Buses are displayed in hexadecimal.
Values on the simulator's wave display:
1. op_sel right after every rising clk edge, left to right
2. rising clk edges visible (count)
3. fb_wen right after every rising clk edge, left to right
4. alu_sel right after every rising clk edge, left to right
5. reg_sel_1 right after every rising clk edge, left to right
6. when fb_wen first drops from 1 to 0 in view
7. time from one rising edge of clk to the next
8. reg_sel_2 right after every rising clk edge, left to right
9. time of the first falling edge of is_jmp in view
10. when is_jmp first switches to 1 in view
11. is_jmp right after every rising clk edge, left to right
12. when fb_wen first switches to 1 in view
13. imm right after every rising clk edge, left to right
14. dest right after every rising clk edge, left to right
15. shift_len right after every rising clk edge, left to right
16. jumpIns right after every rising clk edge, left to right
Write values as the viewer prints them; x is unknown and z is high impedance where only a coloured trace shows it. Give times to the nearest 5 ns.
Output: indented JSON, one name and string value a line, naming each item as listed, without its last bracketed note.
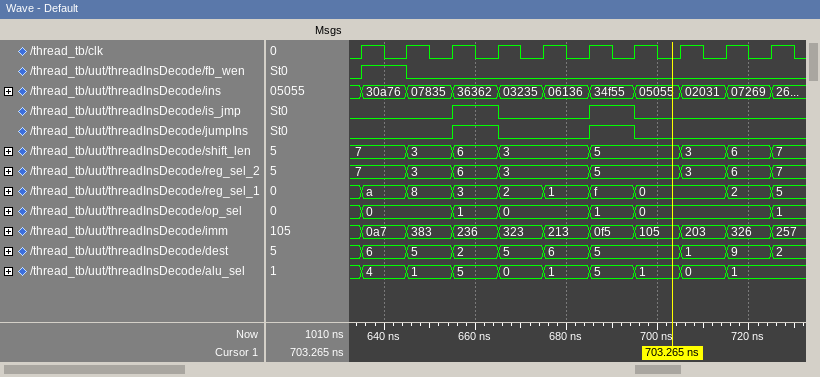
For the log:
{
  "op_sel right after every rising clk edge, left to right": "0, 0, 1, 0, 0, 1, 0, 0, 0, 1",
  "rising clk edges visible": "10",
  "fb_wen right after every rising clk edge, left to right": "1 0 0 0 0 0 0 0 0 0",
  "alu_sel right after every rising clk edge, left to right": "4, 1, 5, 0, 1, 5, 1, 0, 1, 1",
  "reg_sel_1 right after every rising clk edge, left to right": "a, 8, 3, 2, 1, f, 0, 0, 2, 5",
  "when fb_wen first drops from 1 to 0 in view": "645 ns",
  "time from one rising edge of clk to the next": "10 ns",
  "reg_sel_2 right after every rising clk edge, left to right": "7, 3, 6, 3, 3, 5, 5, 3, 6, 7",
  "time of the first falling edge of is_jmp in view": "665 ns",
  "when is_jmp first switches to 1 in view": "655 ns",
  "is_jmp right after every rising clk edge, left to right": "0 0 1 0 0 1 0 0 0 0",
  "when fb_wen first switches to 1 in view": "635 ns",
  "imm right after every rising clk edge, left to right": "0a7, 383, 236, 323, 213, 0f5, 105, 203, 326, 257",
  "dest right after every rising clk edge, left to right": "6, 5, 2, 5, 6, 5, 5, 1, 9, 2",
  "shift_len right after every rising clk edge, left to right": "7, 3, 6, 3, 3, 5, 5, 3, 6, 7",
  "jumpIns right after every rising clk edge, left to right": "0 0 1 0 0 1 0 0 0 0"
}
